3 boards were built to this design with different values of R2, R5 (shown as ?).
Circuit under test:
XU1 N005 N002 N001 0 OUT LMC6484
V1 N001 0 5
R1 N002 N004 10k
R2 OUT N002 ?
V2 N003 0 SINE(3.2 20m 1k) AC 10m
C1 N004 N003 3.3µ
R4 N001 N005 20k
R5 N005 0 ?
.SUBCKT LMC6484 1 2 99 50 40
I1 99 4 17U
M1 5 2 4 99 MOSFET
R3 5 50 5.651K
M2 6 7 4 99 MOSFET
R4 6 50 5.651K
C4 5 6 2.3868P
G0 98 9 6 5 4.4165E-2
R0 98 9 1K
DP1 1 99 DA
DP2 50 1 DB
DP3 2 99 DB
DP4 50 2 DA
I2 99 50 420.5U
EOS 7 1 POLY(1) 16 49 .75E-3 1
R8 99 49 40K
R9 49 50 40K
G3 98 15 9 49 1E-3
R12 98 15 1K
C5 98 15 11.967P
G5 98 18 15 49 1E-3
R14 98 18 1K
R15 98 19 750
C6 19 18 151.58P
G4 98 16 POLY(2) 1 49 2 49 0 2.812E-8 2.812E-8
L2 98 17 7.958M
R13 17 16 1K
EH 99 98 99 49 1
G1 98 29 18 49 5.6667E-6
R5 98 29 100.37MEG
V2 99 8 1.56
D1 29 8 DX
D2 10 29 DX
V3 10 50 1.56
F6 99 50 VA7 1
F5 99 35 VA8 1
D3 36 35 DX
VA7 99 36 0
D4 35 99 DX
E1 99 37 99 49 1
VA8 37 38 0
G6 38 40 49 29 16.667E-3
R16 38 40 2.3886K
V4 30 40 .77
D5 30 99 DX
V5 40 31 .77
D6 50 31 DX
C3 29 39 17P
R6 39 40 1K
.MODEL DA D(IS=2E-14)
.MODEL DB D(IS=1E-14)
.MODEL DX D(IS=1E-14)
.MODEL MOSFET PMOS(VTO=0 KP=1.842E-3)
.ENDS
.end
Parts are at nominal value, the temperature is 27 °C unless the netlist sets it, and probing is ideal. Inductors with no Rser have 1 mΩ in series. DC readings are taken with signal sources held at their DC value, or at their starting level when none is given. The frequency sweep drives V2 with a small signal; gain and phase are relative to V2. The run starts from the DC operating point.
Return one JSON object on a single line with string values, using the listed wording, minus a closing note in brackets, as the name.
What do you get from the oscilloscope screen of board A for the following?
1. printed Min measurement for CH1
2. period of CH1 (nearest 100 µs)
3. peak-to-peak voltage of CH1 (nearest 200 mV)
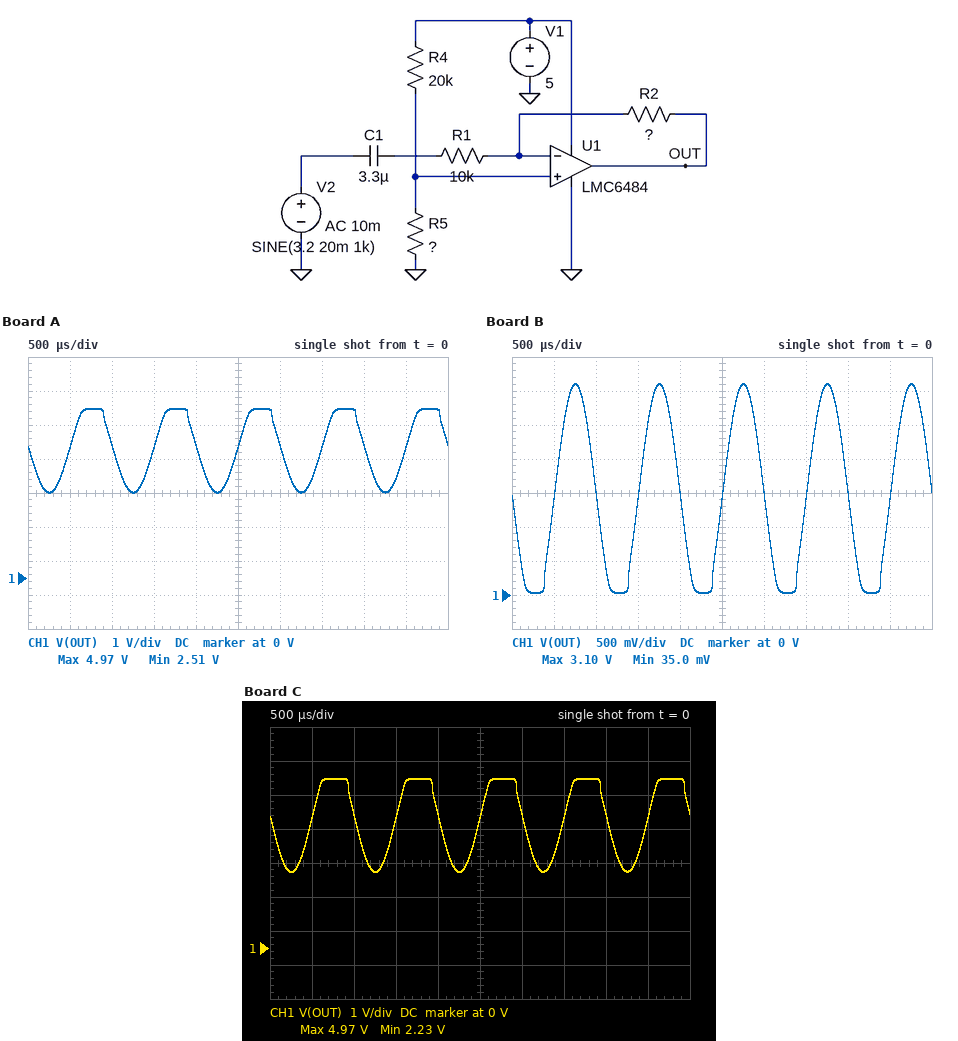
{"printed Min measurement for CH1": "2.51 V", "period of CH1": "1.0 ms", "peak-to-peak voltage of CH1": "2.4 V"}
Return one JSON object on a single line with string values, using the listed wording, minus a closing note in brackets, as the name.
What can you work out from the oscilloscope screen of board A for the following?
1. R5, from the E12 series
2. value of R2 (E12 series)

{"R5, from the E12 series": "68 kΩ", "value of R2": "680 kΩ"}
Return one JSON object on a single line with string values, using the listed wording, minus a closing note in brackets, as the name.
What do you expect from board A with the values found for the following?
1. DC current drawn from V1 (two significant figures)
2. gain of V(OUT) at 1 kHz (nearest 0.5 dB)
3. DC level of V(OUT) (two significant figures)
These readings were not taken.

{"DC current drawn from V1": "560 µA", "gain of V(OUT) at 1 kHz": "36.5 dB", "DC level of V(OUT)": "3.9 V"}
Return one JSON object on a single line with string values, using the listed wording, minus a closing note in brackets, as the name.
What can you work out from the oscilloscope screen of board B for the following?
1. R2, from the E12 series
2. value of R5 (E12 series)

{"R2, from the E12 series": "820 kΩ", "value of R5": "8.2 kΩ"}
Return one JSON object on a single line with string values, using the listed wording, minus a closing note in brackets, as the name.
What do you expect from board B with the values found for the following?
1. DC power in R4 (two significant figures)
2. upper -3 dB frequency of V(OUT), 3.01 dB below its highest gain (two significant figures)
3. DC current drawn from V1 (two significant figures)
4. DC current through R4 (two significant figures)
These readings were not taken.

{"DC power in R4": "630 µW", "upper -3 dB frequency of V(OUT), 3.01 dB below its highest gain": "28 kHz", "DC current drawn from V1": "680 µA", "DC current through R4": "180 µA"}
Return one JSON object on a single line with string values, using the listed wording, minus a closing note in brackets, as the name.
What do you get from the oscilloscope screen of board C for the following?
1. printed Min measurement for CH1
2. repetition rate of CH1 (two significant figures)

{"printed Min measurement for CH1": "2.23 V", "repetition rate of CH1": "1.0 kHz"}
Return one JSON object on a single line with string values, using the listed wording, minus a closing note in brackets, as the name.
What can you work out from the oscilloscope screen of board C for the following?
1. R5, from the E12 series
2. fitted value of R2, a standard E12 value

{"R5, from the E12 series": "68 kΩ", "fitted value of R2, a standard E12 value": "820 kΩ"}
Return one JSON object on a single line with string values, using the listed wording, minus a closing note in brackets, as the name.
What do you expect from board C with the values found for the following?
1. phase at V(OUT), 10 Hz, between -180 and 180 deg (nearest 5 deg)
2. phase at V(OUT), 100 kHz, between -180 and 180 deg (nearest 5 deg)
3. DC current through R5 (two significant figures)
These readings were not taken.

{"phase at V(OUT), 10 Hz, between -180 and 180 deg": "-155 deg", "phase at V(OUT), 100 kHz, between -180 and 180 deg": "100 deg", "DC current through R5": "57 µA"}
